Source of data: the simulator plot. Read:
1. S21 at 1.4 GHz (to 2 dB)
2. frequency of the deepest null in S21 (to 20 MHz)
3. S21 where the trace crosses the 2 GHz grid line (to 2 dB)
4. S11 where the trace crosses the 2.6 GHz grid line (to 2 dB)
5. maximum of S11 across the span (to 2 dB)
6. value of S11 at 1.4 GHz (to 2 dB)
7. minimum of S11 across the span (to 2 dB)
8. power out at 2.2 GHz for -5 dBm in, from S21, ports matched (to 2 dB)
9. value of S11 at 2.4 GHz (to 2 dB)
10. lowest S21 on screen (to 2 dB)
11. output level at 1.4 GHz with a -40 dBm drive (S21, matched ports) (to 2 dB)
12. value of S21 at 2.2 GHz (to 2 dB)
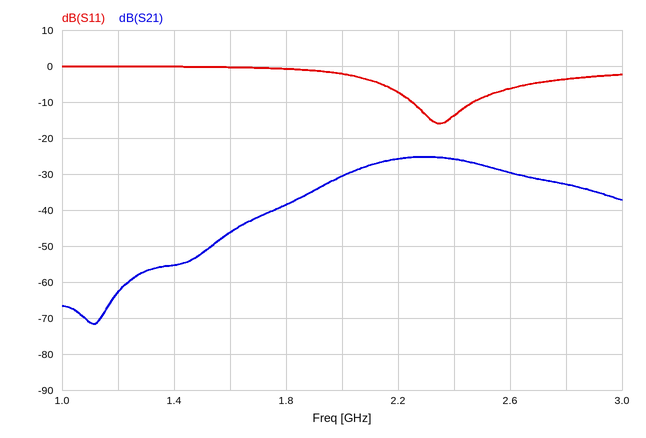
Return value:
-56 dB
1.12 GHz
-30 dB
-6 dB
0 dB
0 dB
-16 dB
-30 dBm
-14 dB
-72 dB
-96 dBm
-26 dB
